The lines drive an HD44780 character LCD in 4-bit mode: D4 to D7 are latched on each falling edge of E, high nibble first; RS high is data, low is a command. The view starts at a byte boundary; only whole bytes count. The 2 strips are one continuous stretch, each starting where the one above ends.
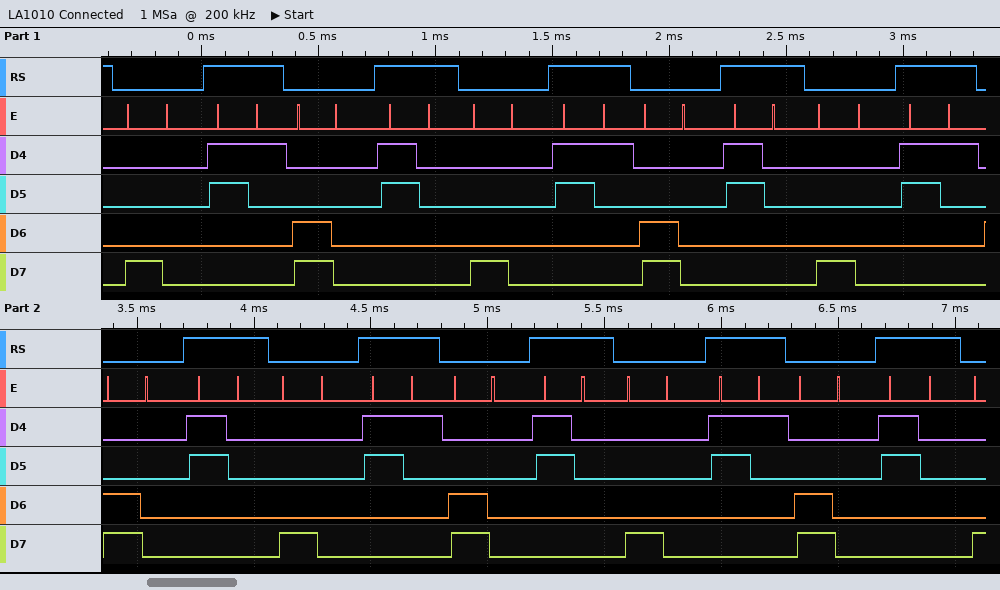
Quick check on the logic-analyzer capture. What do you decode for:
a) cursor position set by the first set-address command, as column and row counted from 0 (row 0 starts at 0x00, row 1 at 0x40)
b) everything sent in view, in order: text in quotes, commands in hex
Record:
column 0, row 0
0x80 "1" 0xC0 "0" 0x80 "1" 0xC0 "0" 0x80 "1" 0xC0 "0" 0x80 "1" 0xC0 "0" 0x80 "1" 0xC0 "0"
